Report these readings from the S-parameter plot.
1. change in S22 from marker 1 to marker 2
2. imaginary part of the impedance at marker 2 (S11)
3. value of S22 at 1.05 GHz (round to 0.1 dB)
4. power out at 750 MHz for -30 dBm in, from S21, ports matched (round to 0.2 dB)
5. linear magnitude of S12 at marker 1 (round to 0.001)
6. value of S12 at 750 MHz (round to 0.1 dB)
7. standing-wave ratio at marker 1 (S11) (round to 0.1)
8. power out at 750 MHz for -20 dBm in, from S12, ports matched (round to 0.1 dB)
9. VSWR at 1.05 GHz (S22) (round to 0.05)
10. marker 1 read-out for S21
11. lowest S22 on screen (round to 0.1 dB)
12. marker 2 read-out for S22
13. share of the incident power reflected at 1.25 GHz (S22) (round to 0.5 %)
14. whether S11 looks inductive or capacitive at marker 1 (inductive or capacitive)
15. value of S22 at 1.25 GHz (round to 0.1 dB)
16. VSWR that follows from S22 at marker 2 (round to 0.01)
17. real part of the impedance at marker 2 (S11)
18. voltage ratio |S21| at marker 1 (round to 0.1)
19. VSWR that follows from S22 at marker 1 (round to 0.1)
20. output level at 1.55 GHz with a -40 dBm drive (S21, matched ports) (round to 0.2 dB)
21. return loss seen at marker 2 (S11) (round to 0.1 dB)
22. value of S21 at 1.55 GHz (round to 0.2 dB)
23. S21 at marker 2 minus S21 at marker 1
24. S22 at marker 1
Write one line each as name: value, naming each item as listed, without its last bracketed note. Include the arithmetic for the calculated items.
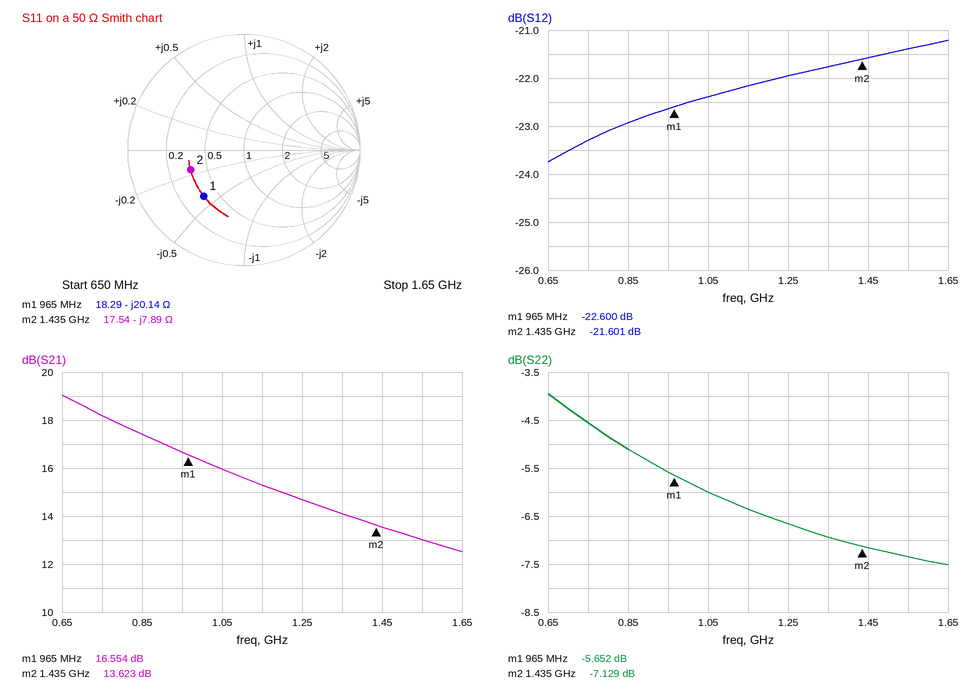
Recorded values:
change in S22 from marker 1 to marker 2: -7.129 − (-5.652) = -1.477 dB
imaginary part of the impedance at marker 2: -7.89 Ω
value of S22 at 1.05 GHz: -6.0 dB
power out at 750 MHz for -30 dBm in, from S21, ports matched: -30 dBm + (18.2 dB) = -11.8 dBm
linear magnitude of S12 at marker 1: 10^(-22.6/20) ≈ 0.074
value of S12 at 750 MHz: -23.3 dB
standing-wave ratio at marker 1 (S11): 3.2
power out at 750 MHz for -20 dBm in, from S12, ports matched: -20 dBm + (-23.3 dB) = -43.3 dBm
VSWR at 1.05 GHz (S22): |Γ| = 10^(-6/20) = 0.5012; VSWR = (1 + 0.5012)/(1 − 0.5012) ≈ 3.01, so 3.00 to the nearest 0.05
marker 1 read-out for S21: 16.554 dB
lowest S22 on screen: -7.5 dB
marker 2 read-out for S22: -7.129 dB
share of the incident power reflected at 1.25 GHz (S22): 10^(-6.7/10) ≈ 21.4 %, so 21.5 % to the nearest 0.5 %
whether S11 looks inductive or capacitive at marker 1: capacitive
value of S22 at 1.25 GHz: -6.7 dB
VSWR that follows from S22 at marker 2: (1 + 0.4401)/(1 − 0.4401) ≈ 2.57
real part of the impedance at marker 2: 17.54 Ω
voltage ratio |S21| at marker 1: 10^(16.554/20) ≈ 6.7
VSWR that follows from S22 at marker 1: (1 + 0.5217)/(1 − 0.5217) ≈ 3.2
output level at 1.55 GHz with a -40 dBm drive (S21, matched ports): -40 dBm + (13.0 dB) = -27.0 dBm
return loss seen at marker 2 (S11): 6.2 dB
value of S21 at 1.55 GHz: 13.0 dB
S21 at marker 2 minus S21 at marker 1: 13.623 − (16.554) = -2.931 dB
S22 at marker 1: -5.652 dB
